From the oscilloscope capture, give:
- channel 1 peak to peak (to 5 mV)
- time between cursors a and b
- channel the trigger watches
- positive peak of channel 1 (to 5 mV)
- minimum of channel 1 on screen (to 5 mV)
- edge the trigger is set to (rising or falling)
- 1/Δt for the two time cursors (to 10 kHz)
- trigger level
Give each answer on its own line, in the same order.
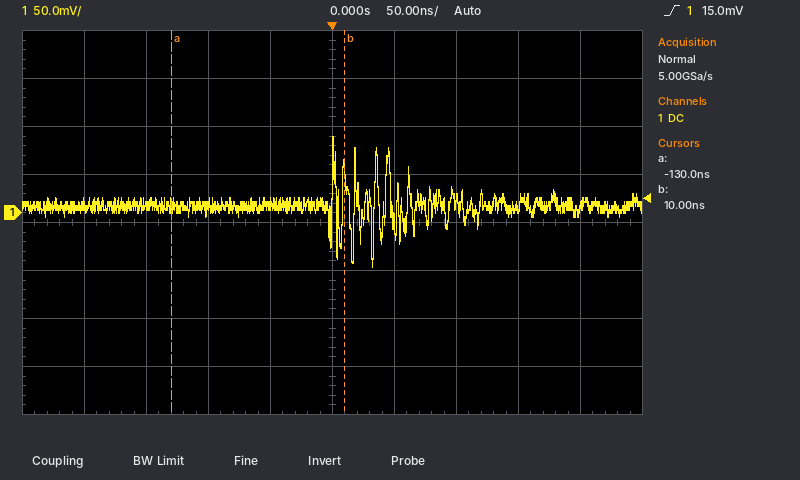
135 mV
140 ns
channel 1
80 mV
-55 mV
rising
7.14 MHz
15.0 mV
